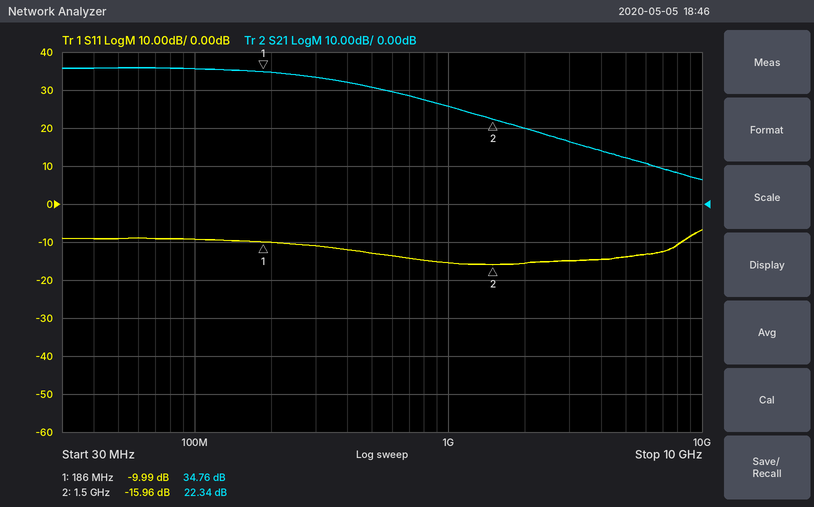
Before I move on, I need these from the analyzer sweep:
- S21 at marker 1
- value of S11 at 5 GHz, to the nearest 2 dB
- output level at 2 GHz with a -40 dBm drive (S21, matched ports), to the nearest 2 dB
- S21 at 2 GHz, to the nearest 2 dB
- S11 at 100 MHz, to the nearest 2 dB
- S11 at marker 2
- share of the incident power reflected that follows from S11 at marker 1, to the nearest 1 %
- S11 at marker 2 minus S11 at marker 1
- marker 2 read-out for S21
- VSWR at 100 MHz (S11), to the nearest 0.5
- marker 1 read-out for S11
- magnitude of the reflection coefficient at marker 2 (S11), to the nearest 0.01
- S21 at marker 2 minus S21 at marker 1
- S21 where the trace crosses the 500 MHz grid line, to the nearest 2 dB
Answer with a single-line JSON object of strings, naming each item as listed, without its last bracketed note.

{"S21 at marker 1": "34.76 dB", "value of S11 at 5 GHz, to the nearest 2 dB": "-14 dB", "output level at 2 GHz with a -40 dBm drive (S21, matched ports), to the nearest 2 dB": "-20 dBm", "S21 at 2 GHz, to the nearest 2 dB": "20 dB", "S11 at 100 MHz, to the nearest 2 dB": "-10 dB", "S11 at marker 2": "-15.96 dB", "share of the incident power reflected that follows from S11 at marker 1, to the nearest 1 %": "10 %", "S11 at marker 2 minus S11 at marker 1": "-5.97 dB", "marker 2 read-out for S21": "22.34 dB", "VSWR at 100 MHz (S11), to the nearest 0.5": "2.0", "marker 1 read-out for S11": "-9.99 dB", "magnitude of the reflection coefficient at marker 2 (S11), to the nearest 0.01": "0.16", "S21 at marker 2 minus S21 at marker 1": "-12.42 dB", "S21 where the trace crosses the 500 MHz grid line, to the nearest 2 dB": "30 dB"}
